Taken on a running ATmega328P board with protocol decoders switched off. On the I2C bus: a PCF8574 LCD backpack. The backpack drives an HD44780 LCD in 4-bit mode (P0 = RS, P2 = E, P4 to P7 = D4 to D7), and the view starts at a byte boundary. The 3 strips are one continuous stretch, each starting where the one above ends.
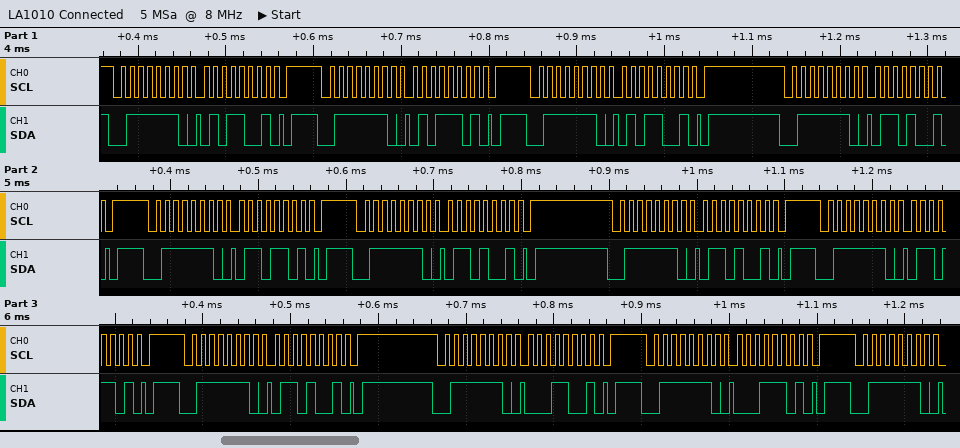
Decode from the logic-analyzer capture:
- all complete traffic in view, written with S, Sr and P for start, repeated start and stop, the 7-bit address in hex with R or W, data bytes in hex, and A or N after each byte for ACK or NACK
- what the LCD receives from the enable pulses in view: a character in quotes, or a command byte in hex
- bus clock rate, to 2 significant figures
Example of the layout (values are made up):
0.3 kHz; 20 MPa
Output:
S 3FW A 59 A P S 3FW A 5D A P S 3FW A 59 A P S 3FW A 69 A P S 3FW A 6D A P S 3FW A 69 A P S 3FW A 69 A P S 3FW A 6D A P S 3FW A 69 A P S 3FW A 19 A P S 3FW A 1D A P S 3FW A; 'V'; 100 kHz
